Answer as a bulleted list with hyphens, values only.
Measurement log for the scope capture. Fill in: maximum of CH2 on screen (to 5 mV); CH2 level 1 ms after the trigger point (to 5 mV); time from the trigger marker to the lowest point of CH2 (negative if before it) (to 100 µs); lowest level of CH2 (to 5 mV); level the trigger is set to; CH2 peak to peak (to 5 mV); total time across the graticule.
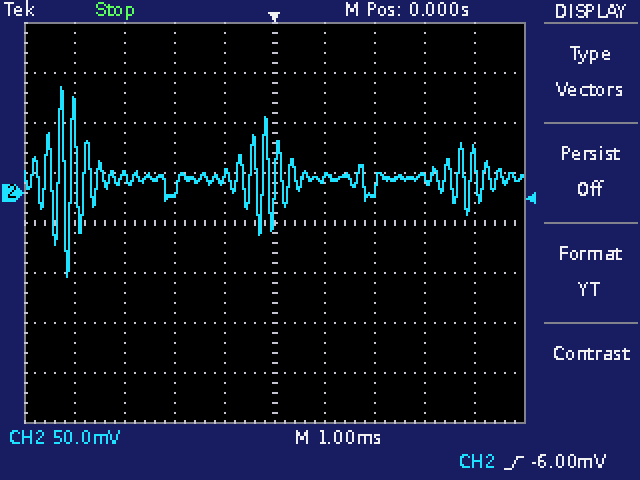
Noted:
- 105 mV
- 15 mV
- -4.1 ms
- -85 mV
- -6.00 mV
- 190 mV
- 10 ms
